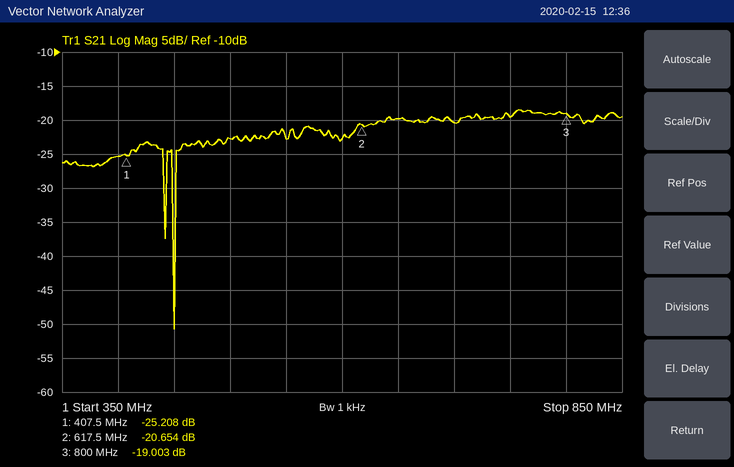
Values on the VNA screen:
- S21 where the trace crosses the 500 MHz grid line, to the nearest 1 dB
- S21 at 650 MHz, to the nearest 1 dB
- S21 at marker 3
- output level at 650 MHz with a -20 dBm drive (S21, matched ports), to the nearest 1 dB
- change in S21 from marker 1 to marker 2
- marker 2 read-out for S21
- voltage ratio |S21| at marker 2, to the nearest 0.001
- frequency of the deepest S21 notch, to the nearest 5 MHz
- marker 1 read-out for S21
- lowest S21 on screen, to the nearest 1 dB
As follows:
-23 dB
-20 dB
-19.003 dB
-40 dBm
4.554 dB
-20.654 dB
0.093
450 MHz
-25.208 dB
-51 dB
